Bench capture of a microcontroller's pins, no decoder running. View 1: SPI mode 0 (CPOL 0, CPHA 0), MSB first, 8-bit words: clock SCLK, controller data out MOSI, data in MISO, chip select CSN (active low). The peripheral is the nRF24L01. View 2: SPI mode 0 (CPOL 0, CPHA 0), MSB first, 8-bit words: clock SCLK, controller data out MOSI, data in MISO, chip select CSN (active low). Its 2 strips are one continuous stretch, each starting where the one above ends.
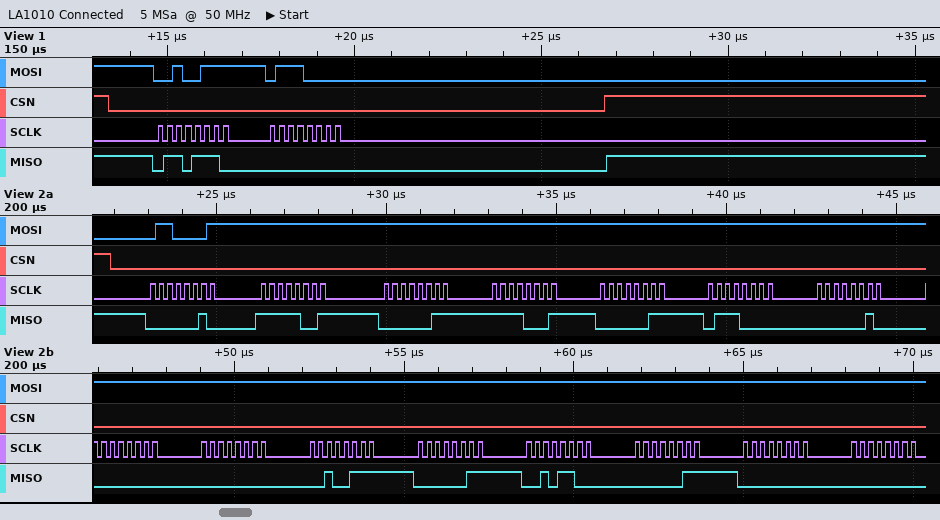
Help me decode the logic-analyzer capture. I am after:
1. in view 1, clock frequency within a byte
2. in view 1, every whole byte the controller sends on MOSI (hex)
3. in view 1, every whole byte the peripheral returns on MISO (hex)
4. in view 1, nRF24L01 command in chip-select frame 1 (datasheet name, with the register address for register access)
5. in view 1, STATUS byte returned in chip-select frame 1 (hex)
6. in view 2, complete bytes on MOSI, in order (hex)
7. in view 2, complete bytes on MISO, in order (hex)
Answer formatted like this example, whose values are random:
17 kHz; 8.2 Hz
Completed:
4 MHz; 27 70; 6E 00; W_REGISTER 0x07; 0x6E; 61 FF FF FF FF FF FF FF FF FF FF FF FF FF FF; 02 F9 03 F1 03 70 02 00 00 27 03 2C 03 00 00
